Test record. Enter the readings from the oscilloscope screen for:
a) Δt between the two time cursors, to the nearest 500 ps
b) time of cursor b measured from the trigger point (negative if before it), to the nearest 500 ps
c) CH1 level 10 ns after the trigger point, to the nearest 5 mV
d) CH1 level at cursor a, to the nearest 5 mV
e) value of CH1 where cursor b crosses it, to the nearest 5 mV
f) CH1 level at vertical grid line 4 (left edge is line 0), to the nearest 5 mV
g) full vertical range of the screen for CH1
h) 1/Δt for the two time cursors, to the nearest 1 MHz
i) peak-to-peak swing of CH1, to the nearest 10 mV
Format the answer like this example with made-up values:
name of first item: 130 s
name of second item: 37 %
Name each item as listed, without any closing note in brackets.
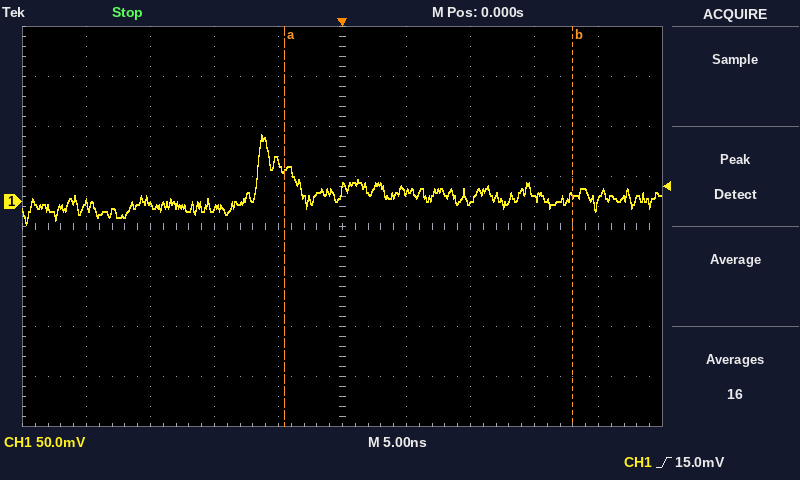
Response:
Δt between the two time cursors, to the nearest 500 ps: 22.5 ns
time of cursor b measured from the trigger point (negative if before it), to the nearest 500 ps: +18.0 ns
CH1 level 10 ns after the trigger point, to the nearest 5 mV: 0 mV
CH1 level at cursor a, to the nearest 5 mV: 30 mV
value of CH1 where cursor b crosses it, to the nearest 5 mV: 5 mV
CH1 level at vertical grid line 4 (left edge is line 0), to the nearest 5 mV: 40 mV
full vertical range of the screen for CH1: 400 mV
1/Δt for the two time cursors, to the nearest 1 MHz: 44 MHz
peak-to-peak swing of CH1, to the nearest 10 mV: 90 mV
